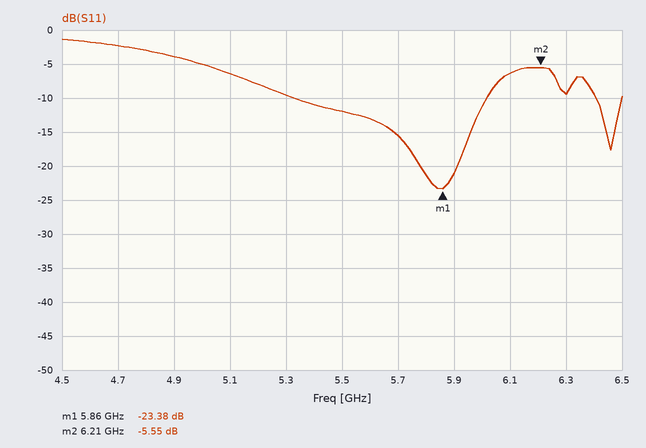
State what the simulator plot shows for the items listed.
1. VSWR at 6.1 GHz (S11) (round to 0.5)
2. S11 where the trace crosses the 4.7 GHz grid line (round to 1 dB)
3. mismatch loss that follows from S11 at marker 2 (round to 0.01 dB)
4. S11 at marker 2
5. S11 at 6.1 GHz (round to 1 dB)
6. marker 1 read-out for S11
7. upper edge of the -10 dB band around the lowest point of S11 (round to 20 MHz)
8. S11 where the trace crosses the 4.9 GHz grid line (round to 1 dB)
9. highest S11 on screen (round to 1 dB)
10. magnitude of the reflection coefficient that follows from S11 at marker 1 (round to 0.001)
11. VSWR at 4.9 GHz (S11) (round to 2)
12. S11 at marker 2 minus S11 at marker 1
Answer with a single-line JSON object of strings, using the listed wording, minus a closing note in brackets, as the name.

{"VSWR at 6.1 GHz (S11)": "3.0", "S11 where the trace crosses the 4.7 GHz grid line": "-2 dB", "mismatch loss that follows from S11 at marker 2": "1.42 dB", "S11 at marker 2": "-5.55 dB", "S11 at 6.1 GHz": "-6 dB", "marker 1 read-out for S11": "-23.38 dB", "upper edge of the -10 dB band around the lowest point of S11": "6.02 GHz", "S11 where the trace crosses the 4.9 GHz grid line": "-4 dB", "highest S11 on screen": "-1 dB", "magnitude of the reflection coefficient that follows from S11 at marker 1": "0.068", "VSWR at 4.9 GHz (S11)": "4", "S11 at marker 2 minus S11 at marker 1": "17.83 dB"}
